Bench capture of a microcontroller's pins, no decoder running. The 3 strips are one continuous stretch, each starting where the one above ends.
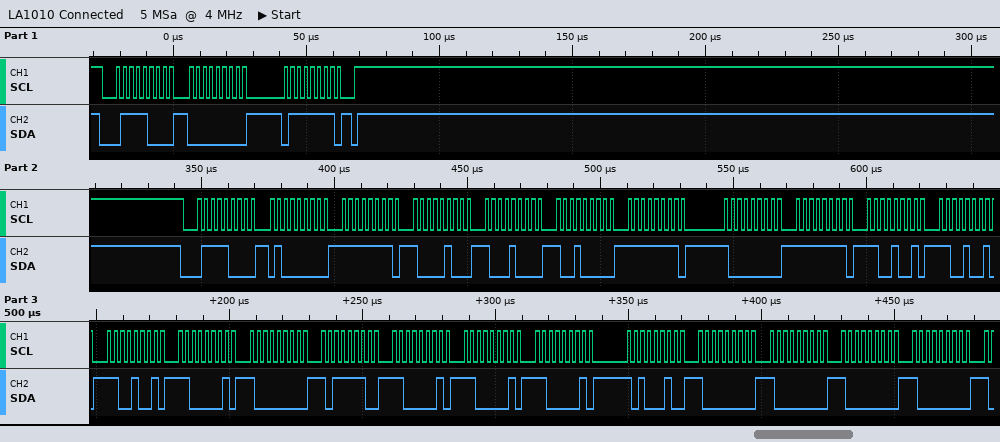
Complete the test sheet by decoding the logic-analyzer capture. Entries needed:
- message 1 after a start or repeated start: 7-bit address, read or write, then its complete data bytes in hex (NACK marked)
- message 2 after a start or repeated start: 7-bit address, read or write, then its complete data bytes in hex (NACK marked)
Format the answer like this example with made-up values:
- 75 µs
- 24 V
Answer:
- 0x3C write: 00 7F
- 0x3C write: 40 FF 84 88 90 FF 80 FF C9 C9 C9 C1 80 BE C1 C1 C1 A2 80 80 80 80
